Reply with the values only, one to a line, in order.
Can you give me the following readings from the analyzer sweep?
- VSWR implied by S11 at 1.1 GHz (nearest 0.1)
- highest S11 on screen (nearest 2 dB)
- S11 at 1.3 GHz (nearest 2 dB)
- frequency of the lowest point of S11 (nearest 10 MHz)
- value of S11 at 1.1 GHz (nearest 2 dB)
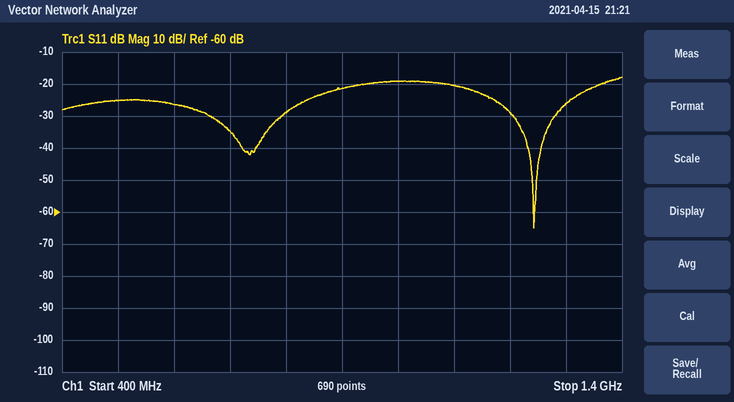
1.2
-18 dB
-26 dB
1.24 GHz
-20 dB
